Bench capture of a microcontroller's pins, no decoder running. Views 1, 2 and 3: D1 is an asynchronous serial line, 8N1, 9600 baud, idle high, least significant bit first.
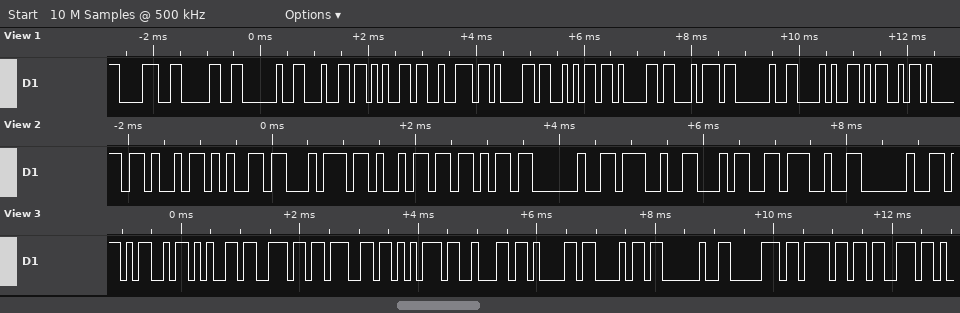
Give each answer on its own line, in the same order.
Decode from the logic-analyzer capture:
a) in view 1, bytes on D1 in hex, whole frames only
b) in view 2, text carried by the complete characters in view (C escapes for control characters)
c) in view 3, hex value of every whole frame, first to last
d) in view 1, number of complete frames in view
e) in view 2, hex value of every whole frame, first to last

38 30 20 64 65 72 61 6A 61 74 20 28 4D
"Ketik '4' "
4D 65 6E 67 75 62 61 68 20 70 6F 73
13
4B 65 74 69 6B 20 27 34 27 20
